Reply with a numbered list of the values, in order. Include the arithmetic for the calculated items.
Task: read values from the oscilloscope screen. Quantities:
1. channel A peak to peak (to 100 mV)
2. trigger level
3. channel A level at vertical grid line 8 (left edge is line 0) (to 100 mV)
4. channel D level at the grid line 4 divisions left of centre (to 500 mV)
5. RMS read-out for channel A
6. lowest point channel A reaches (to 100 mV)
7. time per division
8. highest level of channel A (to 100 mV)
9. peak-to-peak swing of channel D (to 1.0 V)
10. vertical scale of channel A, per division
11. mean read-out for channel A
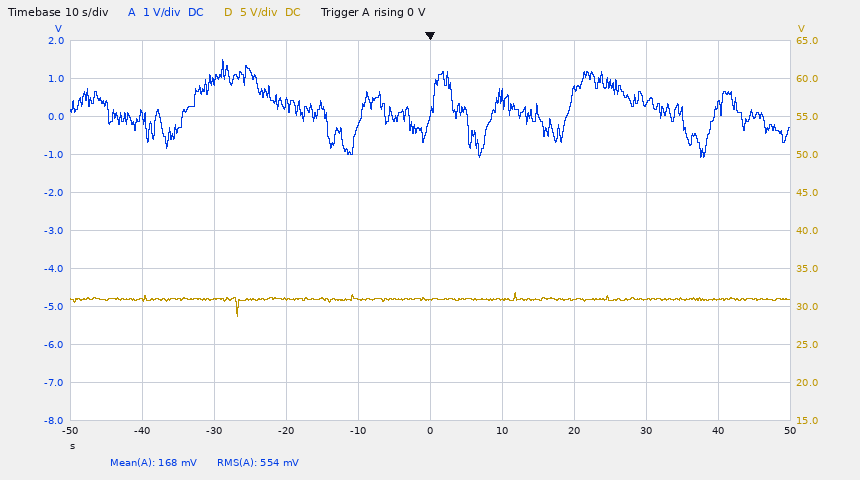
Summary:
1. 1.5 V − (-1.1 V) = 2.6 V
2. 0 V
3. 300 mV
4. 31.0 V
5. 554 mV
6. -1.1 V
7. 10 s
8. 1.5 V
9. 3.0 V
10. 1 V
11. 168 mV
